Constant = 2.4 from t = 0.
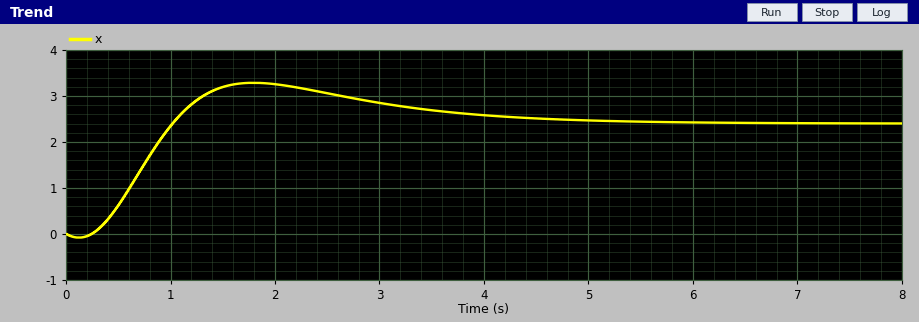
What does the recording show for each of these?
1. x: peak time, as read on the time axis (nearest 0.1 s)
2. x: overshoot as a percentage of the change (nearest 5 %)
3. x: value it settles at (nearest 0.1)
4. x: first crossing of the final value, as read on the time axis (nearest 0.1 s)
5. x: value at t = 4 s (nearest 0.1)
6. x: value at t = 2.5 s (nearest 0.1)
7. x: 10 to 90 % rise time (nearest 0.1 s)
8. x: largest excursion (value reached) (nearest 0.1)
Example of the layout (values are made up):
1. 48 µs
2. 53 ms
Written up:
1. 1.8 s
2. 35 %
3. 2.4
4. 1.0 s
5. 2.6
6. 3.1
7. 0.6 s
8. 3.3
